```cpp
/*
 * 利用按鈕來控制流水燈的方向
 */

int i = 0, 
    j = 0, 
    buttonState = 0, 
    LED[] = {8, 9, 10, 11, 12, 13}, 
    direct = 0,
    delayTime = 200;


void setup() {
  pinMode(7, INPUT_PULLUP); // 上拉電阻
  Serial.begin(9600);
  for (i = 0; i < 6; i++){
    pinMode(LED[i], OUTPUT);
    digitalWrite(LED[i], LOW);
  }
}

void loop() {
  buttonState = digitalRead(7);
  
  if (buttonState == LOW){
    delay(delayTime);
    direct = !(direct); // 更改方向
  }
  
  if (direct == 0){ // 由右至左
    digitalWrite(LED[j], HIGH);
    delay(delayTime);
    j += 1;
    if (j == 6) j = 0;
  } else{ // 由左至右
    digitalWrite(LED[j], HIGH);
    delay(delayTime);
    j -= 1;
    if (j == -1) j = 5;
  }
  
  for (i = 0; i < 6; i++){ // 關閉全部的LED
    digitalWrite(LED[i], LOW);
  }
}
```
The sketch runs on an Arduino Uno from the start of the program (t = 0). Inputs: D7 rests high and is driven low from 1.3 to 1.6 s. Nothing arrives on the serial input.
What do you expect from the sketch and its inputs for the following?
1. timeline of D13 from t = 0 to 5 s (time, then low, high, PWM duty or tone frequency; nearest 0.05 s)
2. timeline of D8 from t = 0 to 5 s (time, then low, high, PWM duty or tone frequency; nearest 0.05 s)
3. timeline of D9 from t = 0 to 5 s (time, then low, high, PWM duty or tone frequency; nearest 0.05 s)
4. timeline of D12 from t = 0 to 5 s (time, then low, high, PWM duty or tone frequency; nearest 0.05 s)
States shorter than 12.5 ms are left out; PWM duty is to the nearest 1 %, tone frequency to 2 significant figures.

0 s low; 1 s high; 1.2 s low; 2 s high; 2.2 s low; 3.2 s high; 3.4 s low; 4.4 s high; 4.6 s low
0 s high; 0.2 s low; 1.2 s high; 1.4 s low; 1.8 s high; 2 s low; 3 s high; 3.2 s low; 4.2 s high; 4.4 s low
0 s low; 0.2 s high; 0.4 s low; 1.6 s high; 1.8 s low; 2.8 s high; 3 s low; 4 s high; 4.2 s low
0 s low; 0.8 s high; 1 s low; 2.2 s high; 2.4 s low; 3.4 s high; 3.6 s low; 4.6 s high; 4.8 s low
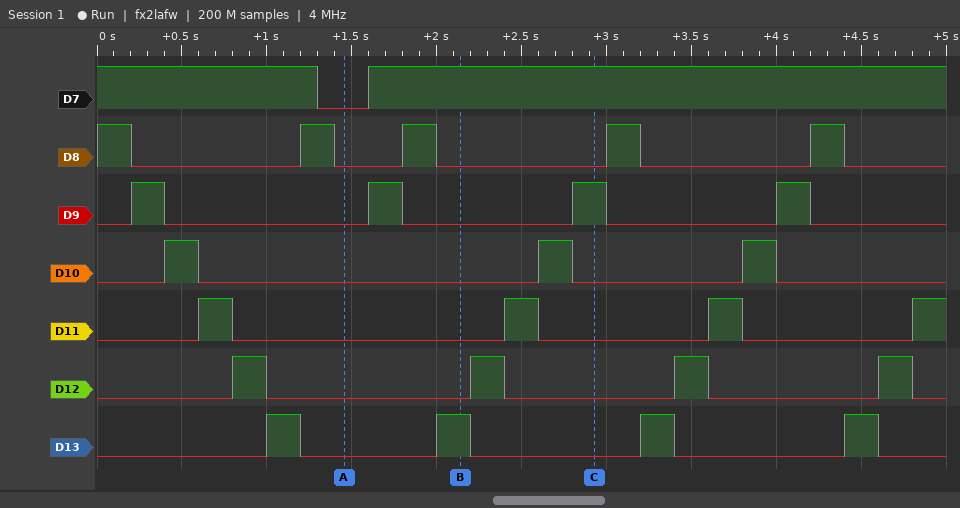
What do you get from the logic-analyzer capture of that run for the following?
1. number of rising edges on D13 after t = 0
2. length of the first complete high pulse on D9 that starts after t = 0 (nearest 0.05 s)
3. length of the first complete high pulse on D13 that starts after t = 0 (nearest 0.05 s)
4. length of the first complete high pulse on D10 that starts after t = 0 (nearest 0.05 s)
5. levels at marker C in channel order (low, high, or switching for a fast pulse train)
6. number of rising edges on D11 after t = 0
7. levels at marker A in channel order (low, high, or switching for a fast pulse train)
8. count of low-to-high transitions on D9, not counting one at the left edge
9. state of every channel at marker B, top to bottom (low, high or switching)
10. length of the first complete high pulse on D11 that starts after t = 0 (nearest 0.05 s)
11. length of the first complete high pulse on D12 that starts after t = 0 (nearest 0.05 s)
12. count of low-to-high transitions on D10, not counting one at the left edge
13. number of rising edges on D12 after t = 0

4
0.20 s
0.20 s
0.20 s
D7 high, D8 low, D9 high, D10 low, D11 low, D12 low, D13 low
4
D7 low, D8 low, D9 low, D10 low, D11 low, D12 low, D13 low
4
D7 high, D8 low, D9 low, D10 low, D11 low, D12 low, D13 high
0.20 s
0.20 s
3
4
